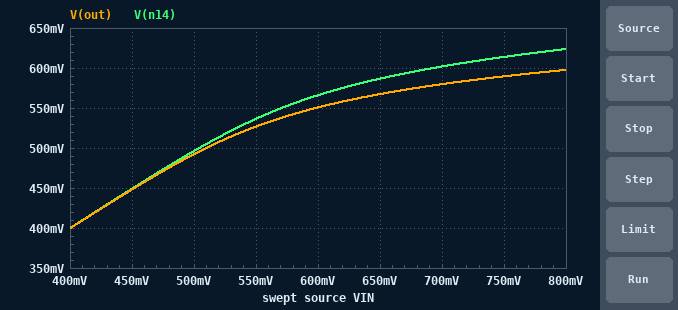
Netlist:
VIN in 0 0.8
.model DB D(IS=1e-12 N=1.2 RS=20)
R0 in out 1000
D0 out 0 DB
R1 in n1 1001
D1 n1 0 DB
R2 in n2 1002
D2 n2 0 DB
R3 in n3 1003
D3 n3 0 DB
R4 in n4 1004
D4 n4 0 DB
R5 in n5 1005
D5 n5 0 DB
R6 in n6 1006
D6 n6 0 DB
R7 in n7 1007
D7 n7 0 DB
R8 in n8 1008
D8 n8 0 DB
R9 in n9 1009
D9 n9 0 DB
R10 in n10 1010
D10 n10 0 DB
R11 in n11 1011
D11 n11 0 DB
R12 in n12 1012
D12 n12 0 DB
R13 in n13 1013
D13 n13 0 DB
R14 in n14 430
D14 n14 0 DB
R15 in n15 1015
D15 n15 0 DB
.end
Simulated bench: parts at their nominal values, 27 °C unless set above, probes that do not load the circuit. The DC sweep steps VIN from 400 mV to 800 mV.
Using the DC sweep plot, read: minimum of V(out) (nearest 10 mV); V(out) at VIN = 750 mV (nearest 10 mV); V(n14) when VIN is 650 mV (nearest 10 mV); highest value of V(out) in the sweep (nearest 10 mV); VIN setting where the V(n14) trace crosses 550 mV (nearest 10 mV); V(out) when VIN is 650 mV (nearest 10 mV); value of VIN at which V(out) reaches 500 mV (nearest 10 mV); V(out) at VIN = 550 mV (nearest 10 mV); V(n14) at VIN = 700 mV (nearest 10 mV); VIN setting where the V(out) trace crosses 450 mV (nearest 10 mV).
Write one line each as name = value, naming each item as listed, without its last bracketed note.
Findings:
minimum of V(out) = 400 mV
V(out) at VIN = 750 mV = 590 mV
V(n14) when VIN is 650 mV = 590 mV
highest value of V(out) in the sweep = 600 mV
VIN setting where the V(n14) trace crosses 550 mV = 570 mV
V(out) when VIN is 650 mV = 570 mV
value of VIN at which V(out) reaches 500 mV = 510 mV
V(out) at VIN = 550 mV = 530 mV
V(n14) at VIN = 700 mV = 600 mV
VIN setting where the V(out) trace crosses 450 mV = 450 mV
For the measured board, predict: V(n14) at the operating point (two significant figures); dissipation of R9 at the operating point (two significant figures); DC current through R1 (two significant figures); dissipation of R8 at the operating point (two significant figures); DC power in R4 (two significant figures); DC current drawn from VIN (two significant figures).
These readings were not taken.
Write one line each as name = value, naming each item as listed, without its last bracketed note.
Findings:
V(n14) at the operating point = 620 mV
dissipation of R9 at the operating point = 41 µW
DC current through R1 = 200 µA
dissipation of R8 at the operating point = 41 µW
DC power in R4 = 41 µW
DC current drawn from VIN = 3.4 mA
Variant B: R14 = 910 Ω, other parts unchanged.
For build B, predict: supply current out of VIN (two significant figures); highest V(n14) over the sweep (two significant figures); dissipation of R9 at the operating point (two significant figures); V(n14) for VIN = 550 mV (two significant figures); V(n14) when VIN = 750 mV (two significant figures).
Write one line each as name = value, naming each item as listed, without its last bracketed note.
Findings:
supply current out of VIN = 3.2 mA
highest V(n14) over the sweep = 600 mV
dissipation of R9 at the operating point = 41 µW
V(n14) for VIN = 550 mV = 530 mV
V(n14) when VIN = 750 mV = 590 mV
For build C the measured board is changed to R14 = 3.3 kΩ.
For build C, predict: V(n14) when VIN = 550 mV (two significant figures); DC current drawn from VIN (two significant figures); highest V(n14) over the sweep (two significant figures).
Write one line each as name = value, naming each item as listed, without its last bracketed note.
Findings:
V(n14) when VIN = 550 mV = 510 mV
DC current drawn from VIN = 3.1 mA
highest V(n14) over the sweep = 560 mV
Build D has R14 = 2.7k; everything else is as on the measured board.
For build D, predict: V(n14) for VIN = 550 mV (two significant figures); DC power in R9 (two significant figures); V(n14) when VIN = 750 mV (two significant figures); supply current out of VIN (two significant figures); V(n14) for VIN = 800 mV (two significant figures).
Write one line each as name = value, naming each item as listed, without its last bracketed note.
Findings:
V(n14) for VIN = 550 mV = 510 mV
DC power in R9 = 41 µW
V(n14) when VIN = 750 mV = 560 mV
supply current out of VIN = 3.1 mA
V(n14) for VIN = 800 mV = 570 mV
